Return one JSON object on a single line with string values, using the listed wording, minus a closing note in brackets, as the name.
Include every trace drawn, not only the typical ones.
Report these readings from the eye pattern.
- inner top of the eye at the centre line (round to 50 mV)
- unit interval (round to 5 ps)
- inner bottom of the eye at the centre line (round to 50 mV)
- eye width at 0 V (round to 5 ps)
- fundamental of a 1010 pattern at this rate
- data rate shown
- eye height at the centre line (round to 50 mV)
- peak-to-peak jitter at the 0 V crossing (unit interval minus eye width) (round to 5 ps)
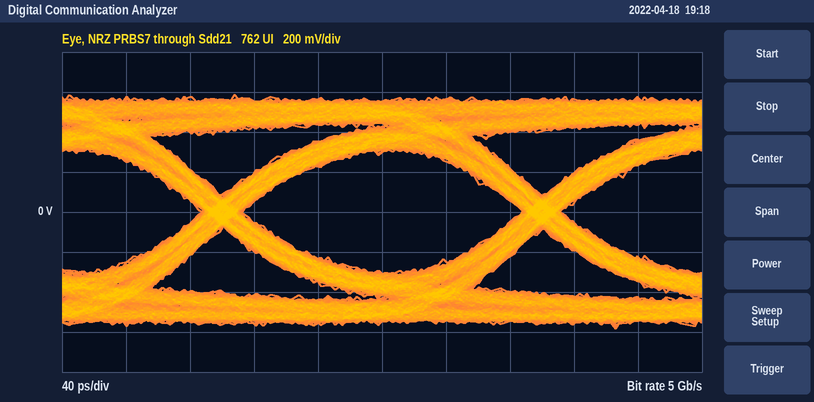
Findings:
{"inner top of the eye at the centre line": "300 mV", "unit interval": "200 ps", "inner bottom of the eye at the centre line": "-300 mV", "eye width at 0 V": "175 ps", "fundamental of a 1010 pattern at this rate": "2.5 GHz", "data rate shown": "5 Gb/s", "eye height at the centre line": "600 mV", "peak-to-peak jitter at the 0 V crossing (unit interval minus eye width)": "25 ps"}
